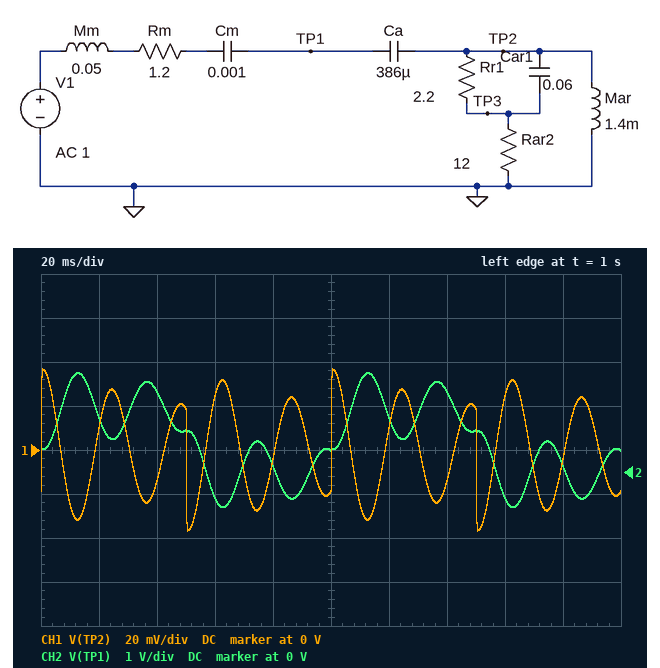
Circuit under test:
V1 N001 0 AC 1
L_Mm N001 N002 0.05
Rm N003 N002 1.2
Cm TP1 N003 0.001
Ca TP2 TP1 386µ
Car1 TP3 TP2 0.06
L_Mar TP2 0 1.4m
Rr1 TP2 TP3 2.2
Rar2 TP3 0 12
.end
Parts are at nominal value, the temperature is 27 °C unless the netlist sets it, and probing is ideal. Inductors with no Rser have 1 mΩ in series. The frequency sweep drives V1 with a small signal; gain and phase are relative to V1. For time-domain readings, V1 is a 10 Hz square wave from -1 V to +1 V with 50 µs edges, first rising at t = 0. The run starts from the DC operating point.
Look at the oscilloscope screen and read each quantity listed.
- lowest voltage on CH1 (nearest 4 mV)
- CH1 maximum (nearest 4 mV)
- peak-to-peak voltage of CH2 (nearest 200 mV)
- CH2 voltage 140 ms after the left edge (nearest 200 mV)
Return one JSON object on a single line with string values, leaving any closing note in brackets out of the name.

{"lowest voltage on CH1": "-36 mV", "CH1 maximum": "36 mV", "peak-to-peak voltage of CH2": "3.0 V", "CH2 voltage 140 ms after the left edge": "1.8 V"}
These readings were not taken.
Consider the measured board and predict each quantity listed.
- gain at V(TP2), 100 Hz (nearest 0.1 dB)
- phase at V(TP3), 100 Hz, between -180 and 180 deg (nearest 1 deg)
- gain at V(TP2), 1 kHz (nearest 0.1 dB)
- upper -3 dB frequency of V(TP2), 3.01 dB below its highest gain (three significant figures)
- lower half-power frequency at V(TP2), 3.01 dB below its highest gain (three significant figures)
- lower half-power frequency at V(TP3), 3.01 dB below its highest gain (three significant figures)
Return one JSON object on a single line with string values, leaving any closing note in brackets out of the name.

{"gain at V(TP2), 100 Hz": "-29.6 dB", "phase at V(TP3), 100 Hz, between -180 and 180 deg": "-1 deg", "gain at V(TP2), 1 kHz": "-33.1 dB", "upper -3 dB frequency of V(TP2), 3.01 dB below its highest gain": "44.2 Hz", "lower half-power frequency at V(TP2), 3.01 dB below its highest gain": "40.4 Hz", "lower half-power frequency at V(TP3), 3.01 dB below its highest gain": "40.4 Hz"}
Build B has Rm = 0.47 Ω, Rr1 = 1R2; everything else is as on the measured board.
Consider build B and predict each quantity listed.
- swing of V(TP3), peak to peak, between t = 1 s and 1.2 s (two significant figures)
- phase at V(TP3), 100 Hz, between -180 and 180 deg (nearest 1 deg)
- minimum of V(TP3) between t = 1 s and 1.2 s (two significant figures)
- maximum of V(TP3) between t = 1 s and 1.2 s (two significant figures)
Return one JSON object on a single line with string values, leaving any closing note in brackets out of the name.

{"swing of V(TP3), peak to peak, between t = 1 s and 1.2 s": "64 mV", "phase at V(TP3), 100 Hz, between -180 and 180 deg": "-3 deg", "minimum of V(TP3) between t = 1 s and 1.2 s": "-32 mV", "maximum of V(TP3) between t = 1 s and 1.2 s": "32 mV"}
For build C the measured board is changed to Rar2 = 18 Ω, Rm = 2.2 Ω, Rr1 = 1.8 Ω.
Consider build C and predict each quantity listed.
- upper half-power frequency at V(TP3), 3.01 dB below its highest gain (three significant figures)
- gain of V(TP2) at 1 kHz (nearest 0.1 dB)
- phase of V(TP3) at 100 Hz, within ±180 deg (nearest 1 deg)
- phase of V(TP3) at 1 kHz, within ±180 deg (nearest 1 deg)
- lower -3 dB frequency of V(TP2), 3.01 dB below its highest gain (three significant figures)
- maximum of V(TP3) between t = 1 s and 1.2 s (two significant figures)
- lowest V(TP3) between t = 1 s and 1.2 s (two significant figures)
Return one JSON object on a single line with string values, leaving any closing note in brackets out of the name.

{"upper half-power frequency at V(TP3), 3.01 dB below its highest gain": "46.3 Hz", "gain of V(TP2) at 1 kHz": "-32.2 dB", "phase of V(TP3) at 100 Hz, within ±180 deg": "2 deg", "phase of V(TP3) at 1 kHz, within ±180 deg": "-25 deg", "lower -3 dB frequency of V(TP2), 3.01 dB below its highest gain": "39.2 Hz", "maximum of V(TP3) between t = 1 s and 1.2 s": "42 mV", "lowest V(TP3) between t = 1 s and 1.2 s": "-42 mV"}
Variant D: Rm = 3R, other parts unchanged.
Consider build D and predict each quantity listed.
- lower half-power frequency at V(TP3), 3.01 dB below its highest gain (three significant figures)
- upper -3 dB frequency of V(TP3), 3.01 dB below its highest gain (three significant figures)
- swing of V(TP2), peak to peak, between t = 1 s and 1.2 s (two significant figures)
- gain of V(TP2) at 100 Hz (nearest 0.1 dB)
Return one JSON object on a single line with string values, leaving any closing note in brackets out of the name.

{"lower half-power frequency at V(TP3), 3.01 dB below its highest gain": "38.5 Hz", "upper -3 dB frequency of V(TP3), 3.01 dB below its highest gain": "48.4 Hz", "swing of V(TP2), peak to peak, between t = 1 s and 1.2 s": "89 mV", "gain of V(TP2) at 100 Hz": "-29.7 dB"}
